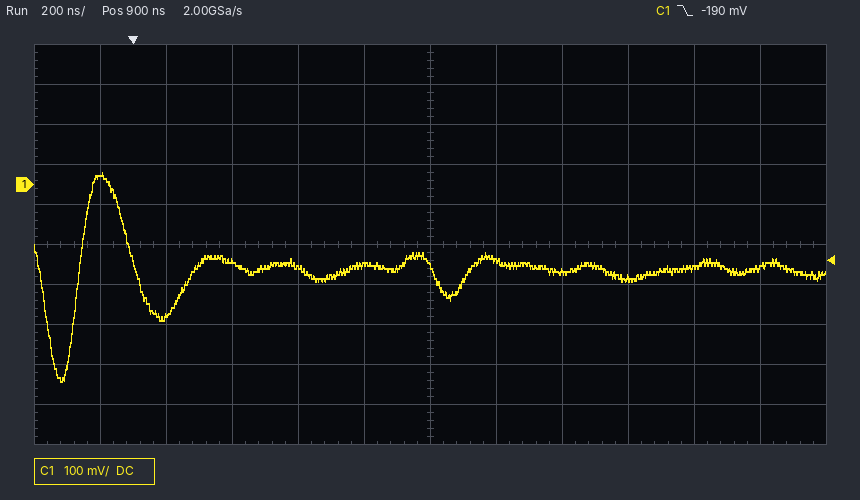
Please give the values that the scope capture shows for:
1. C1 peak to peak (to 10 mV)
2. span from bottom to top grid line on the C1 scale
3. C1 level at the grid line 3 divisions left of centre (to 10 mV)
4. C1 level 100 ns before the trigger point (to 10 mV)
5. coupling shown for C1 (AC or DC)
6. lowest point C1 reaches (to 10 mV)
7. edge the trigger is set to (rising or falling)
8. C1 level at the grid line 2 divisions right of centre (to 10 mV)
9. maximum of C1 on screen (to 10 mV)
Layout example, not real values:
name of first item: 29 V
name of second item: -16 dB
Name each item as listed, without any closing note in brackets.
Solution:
C1 peak to peak: 520 mV
span from bottom to top grid line on the C1 scale: 1 V
C1 level at the grid line 3 divisions left of centre: -190 mV
C1 level 100 ns before the trigger point: 20 mV
coupling shown for C1: DC
lowest point C1 reaches: -490 mV
edge the trigger is set to: falling
C1 level at the grid line 2 divisions right of centre: -220 mV
maximum of C1 on screen: 30 mV
